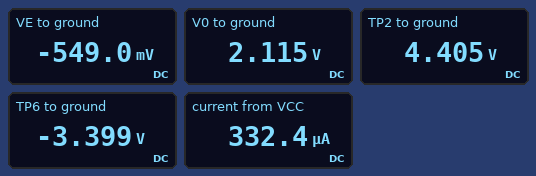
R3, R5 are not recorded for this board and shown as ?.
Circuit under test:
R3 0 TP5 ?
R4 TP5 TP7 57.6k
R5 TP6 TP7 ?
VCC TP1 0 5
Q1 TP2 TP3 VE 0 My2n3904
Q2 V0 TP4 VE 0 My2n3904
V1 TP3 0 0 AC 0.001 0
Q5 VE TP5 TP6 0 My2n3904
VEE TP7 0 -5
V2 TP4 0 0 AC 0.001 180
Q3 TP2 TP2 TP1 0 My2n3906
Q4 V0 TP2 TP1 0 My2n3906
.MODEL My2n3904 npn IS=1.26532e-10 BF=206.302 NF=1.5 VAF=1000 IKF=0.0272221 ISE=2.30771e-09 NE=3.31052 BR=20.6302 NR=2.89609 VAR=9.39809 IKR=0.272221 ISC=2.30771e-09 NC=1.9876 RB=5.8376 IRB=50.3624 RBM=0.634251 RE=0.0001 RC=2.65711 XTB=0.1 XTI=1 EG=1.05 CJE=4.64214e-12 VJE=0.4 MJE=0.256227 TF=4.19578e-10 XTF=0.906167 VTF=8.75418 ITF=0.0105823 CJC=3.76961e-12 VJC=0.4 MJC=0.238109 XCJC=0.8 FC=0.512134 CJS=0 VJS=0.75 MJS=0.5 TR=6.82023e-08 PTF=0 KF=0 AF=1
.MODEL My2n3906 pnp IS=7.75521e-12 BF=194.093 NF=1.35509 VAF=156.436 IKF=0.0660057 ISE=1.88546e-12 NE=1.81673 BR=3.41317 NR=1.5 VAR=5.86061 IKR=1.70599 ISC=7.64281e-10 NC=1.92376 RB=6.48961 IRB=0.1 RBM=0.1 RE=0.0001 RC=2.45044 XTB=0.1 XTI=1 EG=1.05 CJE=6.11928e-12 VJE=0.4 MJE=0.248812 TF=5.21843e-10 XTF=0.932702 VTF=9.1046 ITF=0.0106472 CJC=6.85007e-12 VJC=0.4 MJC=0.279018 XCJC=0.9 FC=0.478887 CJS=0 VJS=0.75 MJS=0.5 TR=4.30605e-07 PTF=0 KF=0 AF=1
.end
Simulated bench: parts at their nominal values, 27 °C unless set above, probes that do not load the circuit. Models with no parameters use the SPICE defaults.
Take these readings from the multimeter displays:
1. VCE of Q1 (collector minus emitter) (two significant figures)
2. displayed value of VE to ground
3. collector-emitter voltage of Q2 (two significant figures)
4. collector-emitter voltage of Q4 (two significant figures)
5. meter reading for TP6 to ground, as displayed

5.0 V
-549.0 mV
2.7 V
-2.9 V
-3.399 V
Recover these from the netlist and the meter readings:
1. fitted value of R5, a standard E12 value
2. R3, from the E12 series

4.7 kΩ
68 kΩ
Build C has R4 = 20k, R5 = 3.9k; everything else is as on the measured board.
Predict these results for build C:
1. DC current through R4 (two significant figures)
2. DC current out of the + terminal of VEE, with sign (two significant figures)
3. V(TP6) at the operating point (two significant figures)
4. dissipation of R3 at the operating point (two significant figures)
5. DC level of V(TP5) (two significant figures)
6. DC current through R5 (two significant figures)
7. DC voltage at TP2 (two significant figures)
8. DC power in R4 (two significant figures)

55 µA
-200 µA
-4.4 V
220 µW
-3.9 V
140 µA
4.4 V
61 µW
